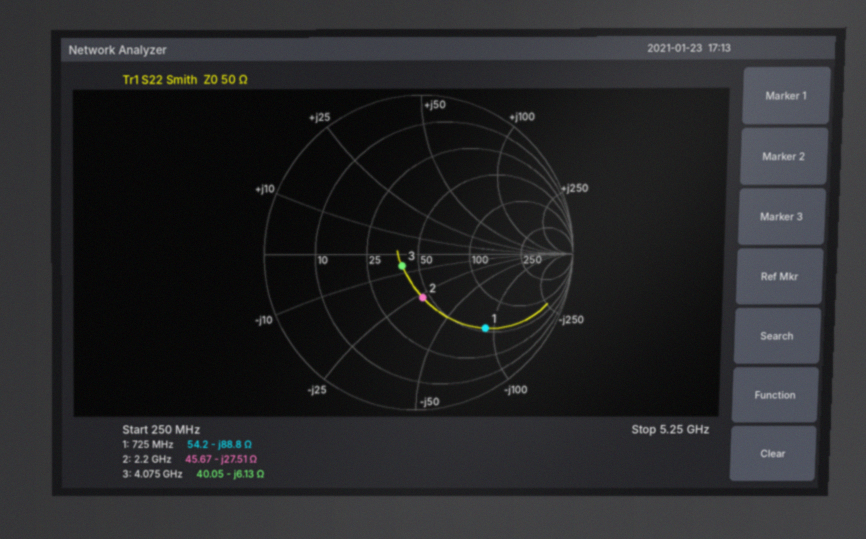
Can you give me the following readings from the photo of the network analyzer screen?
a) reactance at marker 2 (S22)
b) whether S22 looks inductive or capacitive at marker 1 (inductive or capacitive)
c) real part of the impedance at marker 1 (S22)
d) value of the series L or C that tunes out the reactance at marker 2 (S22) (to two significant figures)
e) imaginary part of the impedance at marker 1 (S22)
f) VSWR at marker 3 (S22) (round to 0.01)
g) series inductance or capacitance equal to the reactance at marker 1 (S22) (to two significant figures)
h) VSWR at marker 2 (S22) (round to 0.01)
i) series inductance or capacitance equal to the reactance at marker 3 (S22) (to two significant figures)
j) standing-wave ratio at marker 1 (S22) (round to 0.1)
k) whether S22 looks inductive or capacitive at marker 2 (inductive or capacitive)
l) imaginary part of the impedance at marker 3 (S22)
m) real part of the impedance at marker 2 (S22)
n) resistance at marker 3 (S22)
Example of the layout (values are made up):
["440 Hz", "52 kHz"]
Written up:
["-27.51 Ω", "capacitive", "54.2 Ω", "2.0 nH", "-88.8 Ω", "1.30", "2.5 pF", "1.78", "6.4 pF", "4.7", "capacitive", "-6.13 Ω", "45.67 Ω", "40.05 Ω"]
